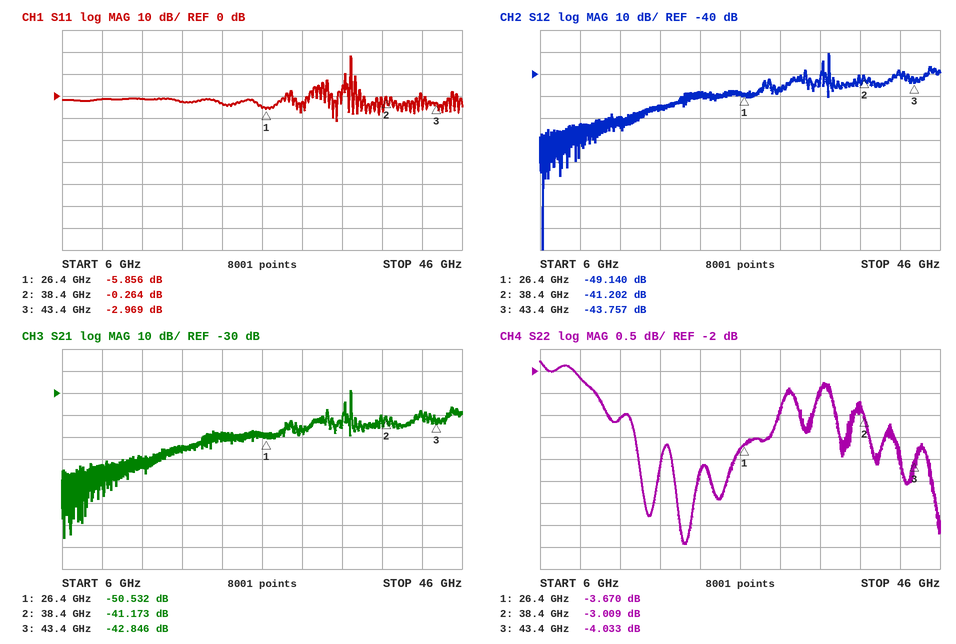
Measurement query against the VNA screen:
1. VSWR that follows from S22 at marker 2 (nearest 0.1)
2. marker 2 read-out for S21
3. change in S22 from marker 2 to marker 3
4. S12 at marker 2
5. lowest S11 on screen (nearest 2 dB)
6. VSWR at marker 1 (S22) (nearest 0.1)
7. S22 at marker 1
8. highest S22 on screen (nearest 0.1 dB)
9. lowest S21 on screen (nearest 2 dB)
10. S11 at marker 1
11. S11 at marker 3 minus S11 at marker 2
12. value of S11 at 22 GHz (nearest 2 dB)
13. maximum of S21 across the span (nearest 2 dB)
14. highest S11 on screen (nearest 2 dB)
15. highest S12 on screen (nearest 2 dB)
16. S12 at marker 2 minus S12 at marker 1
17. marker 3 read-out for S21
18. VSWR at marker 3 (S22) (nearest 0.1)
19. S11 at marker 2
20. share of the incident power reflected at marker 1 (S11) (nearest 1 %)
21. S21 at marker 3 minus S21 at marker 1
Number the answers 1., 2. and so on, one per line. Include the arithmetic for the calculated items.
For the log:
1. (1 + 0.7072)/(1 − 0.7072) ≈ 5.8
2. -41.173 dB
3. -4.033 − (-3.009) = -1.024 dB
4. -41.202 dB
5. -12 dB
6. (1 + 0.6554)/(1 − 0.6554) ≈ 4.8
7. -3.670 dB
8. -1.8 dB
9. -96 dB
10. -5.856 dB
11. -2.969 − (-0.264) = -2.705 dB
12. -4 dB
13. -28 dB
14. 18 dB
15. -30 dB
16. -41.202 − (-49.14) = 7.938 dB
17. -42.846 dB
18. (1 + 0.6286)/(1 − 0.6286) ≈ 4.4
19. -0.264 dB
20. 10^(-5.856/10) ≈ 26 %
21. -42.846 − (-50.532) = 7.686 dB
